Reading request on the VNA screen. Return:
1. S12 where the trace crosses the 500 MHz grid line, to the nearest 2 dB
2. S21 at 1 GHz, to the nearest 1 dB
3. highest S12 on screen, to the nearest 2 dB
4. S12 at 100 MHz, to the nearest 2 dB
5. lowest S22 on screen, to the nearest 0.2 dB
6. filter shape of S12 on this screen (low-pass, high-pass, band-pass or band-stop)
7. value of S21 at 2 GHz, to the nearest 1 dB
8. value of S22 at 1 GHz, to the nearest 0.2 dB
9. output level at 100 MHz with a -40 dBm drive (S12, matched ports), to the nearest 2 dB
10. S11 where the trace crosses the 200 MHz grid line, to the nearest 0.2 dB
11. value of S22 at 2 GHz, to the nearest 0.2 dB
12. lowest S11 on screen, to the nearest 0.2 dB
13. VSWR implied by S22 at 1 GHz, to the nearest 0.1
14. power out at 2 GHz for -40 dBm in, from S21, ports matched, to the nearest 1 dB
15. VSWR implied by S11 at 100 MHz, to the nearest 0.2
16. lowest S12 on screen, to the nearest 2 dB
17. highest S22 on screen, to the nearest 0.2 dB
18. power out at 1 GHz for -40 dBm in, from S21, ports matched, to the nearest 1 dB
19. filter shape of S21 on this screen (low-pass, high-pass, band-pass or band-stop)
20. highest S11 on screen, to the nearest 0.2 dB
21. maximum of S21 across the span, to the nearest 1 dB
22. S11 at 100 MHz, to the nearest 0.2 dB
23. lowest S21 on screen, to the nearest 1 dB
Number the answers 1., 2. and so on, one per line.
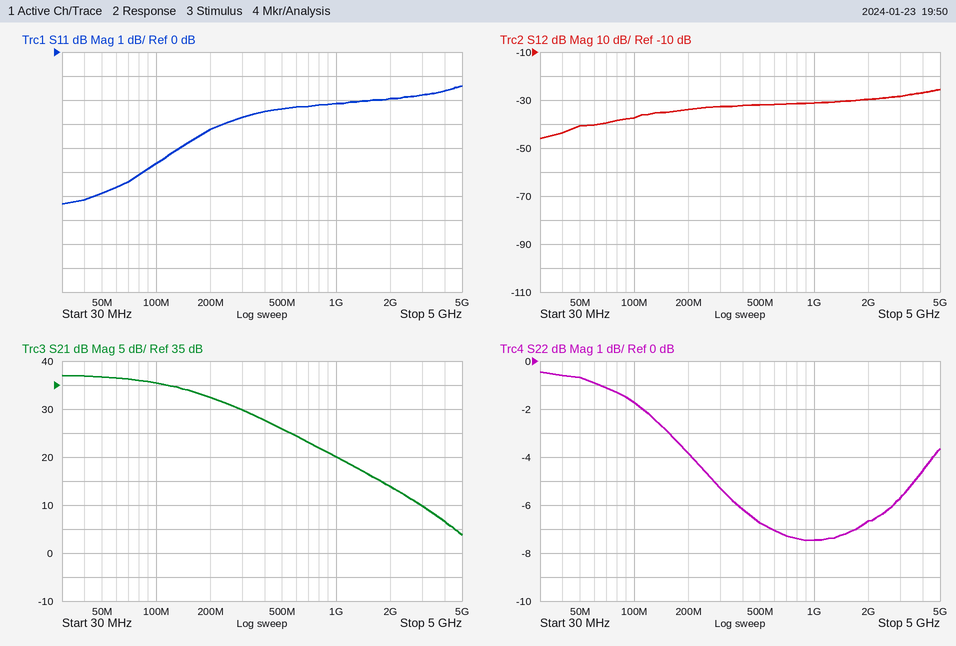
1. -32 dB
2. 20 dB
3. -26 dB
4. -38 dB
5. -7.4 dB
6. high-pass
7. 14 dB
8. -7.4 dB
9. -78 dBm
10. -3.2 dB
11. -6.6 dB
12. -6.4 dB
13. 2.5
14. -26 dBm
15. 3.8
16. -46 dB
17. -0.4 dB
18. -20 dBm
19. low-pass
20. -1.4 dB
21. 37 dB
22. -4.6 dB
23. 4 dB
